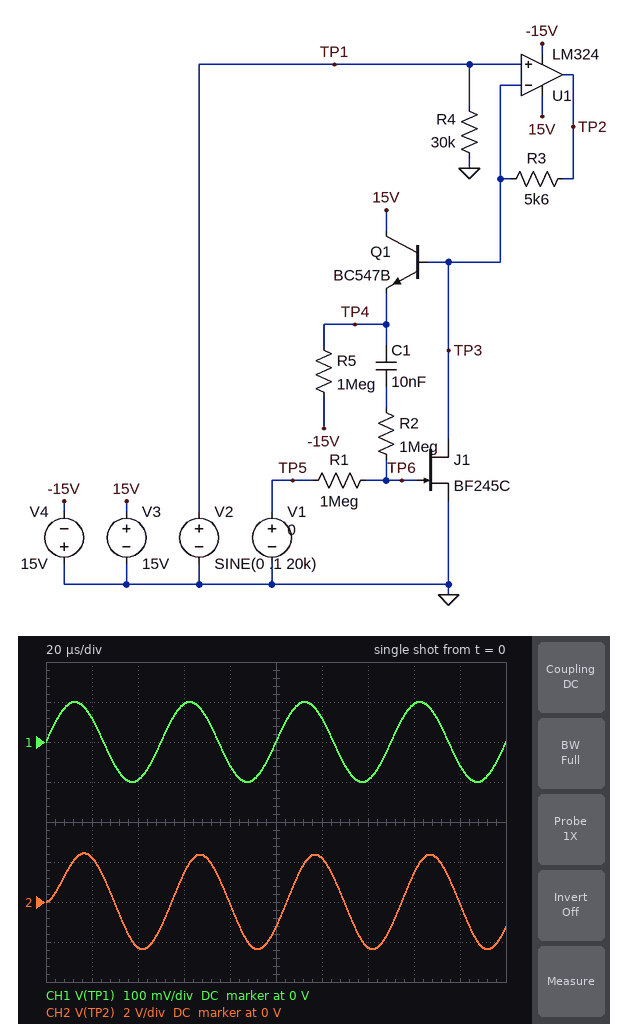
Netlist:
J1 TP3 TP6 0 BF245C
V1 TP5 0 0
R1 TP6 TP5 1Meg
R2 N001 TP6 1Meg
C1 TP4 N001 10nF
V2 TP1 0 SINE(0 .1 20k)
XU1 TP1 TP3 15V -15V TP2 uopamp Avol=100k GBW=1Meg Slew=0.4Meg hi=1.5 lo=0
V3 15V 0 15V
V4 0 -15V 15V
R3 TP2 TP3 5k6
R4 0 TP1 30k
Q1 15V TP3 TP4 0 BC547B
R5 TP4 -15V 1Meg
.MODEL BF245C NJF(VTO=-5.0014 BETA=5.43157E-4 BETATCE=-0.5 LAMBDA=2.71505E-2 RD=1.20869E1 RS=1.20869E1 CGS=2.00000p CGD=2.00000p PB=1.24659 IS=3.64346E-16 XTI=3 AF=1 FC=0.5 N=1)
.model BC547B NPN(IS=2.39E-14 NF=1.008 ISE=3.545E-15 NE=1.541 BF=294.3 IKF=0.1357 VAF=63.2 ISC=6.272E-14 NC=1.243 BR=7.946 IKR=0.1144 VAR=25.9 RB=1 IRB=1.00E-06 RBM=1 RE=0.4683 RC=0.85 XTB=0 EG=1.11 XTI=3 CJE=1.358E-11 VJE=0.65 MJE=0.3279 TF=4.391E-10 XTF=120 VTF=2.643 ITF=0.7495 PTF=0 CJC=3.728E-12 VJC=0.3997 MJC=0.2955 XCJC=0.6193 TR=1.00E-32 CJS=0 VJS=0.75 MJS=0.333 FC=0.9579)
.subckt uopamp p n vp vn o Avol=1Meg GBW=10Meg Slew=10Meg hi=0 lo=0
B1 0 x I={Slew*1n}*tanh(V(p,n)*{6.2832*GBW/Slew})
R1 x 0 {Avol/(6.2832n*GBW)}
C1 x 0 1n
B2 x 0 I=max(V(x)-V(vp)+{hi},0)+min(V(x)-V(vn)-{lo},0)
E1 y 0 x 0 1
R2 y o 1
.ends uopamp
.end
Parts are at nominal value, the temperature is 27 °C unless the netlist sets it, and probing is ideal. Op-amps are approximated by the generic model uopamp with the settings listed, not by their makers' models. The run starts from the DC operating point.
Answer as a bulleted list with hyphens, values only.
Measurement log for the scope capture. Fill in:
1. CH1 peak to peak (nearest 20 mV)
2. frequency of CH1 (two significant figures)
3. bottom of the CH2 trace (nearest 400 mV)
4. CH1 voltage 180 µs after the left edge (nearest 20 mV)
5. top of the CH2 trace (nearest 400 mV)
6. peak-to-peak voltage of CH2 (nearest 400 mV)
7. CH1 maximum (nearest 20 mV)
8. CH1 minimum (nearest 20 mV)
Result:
- 200 mV
- 20 kHz
- -2.4 V
- -60 mV
- 2.4 V
- 4.8 V
- 100 mV
- -100 mV
